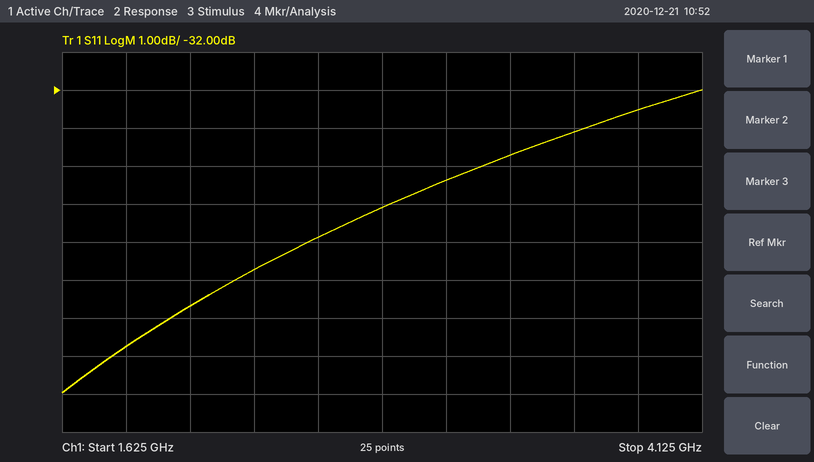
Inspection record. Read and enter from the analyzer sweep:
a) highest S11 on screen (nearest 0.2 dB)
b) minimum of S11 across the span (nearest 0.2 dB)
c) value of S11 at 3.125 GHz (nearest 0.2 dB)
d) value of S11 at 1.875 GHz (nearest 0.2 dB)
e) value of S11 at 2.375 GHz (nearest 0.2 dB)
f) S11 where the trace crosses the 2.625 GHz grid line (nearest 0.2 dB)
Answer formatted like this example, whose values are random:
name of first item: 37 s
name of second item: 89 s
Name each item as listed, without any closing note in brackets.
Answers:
highest S11 on screen: -32.0 dB
minimum of S11 across the span: -40.0 dB
value of S11 at 3.125 GHz: -34.4 dB
value of S11 at 1.875 GHz: -38.8 dB
value of S11 at 2.375 GHz: -36.8 dB
S11 where the trace crosses the 2.625 GHz grid line: -35.8 dB
